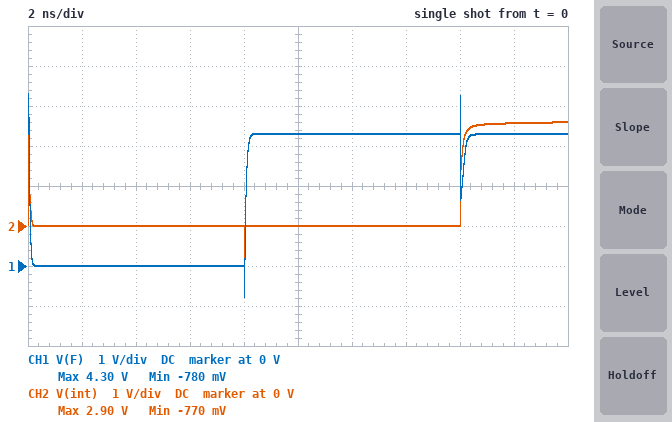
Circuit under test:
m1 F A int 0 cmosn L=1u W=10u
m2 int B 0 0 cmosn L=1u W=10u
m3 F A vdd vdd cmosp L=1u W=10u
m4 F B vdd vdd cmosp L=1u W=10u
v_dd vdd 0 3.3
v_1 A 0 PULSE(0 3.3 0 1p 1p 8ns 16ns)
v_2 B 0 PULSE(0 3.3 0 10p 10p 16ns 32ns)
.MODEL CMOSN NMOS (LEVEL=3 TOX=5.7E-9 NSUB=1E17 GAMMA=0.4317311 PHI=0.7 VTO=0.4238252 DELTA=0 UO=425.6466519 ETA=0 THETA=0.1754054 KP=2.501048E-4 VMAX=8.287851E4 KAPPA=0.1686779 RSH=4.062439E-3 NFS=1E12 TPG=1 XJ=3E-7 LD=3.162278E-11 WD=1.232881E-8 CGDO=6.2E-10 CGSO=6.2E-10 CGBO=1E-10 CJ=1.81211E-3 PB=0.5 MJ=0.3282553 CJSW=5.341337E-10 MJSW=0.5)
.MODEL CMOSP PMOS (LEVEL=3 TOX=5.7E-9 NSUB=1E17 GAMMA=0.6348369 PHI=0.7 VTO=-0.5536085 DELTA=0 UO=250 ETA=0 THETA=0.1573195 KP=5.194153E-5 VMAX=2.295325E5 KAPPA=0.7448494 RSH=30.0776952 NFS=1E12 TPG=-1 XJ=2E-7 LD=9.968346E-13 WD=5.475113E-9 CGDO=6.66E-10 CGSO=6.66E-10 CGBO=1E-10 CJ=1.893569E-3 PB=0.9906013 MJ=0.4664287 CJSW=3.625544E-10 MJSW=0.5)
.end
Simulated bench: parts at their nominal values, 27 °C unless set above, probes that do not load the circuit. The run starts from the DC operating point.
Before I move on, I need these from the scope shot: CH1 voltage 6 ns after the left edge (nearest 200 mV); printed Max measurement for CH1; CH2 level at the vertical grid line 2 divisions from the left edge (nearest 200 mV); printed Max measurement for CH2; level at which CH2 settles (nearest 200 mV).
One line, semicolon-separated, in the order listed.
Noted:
0 V; 4.30 V; 0 V; 2.90 V; 2.6 V
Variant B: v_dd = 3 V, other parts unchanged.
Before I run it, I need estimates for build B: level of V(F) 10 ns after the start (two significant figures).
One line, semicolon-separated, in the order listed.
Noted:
3.0 V
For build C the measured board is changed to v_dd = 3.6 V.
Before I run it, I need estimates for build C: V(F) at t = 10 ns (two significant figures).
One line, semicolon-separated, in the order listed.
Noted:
3.6 V
